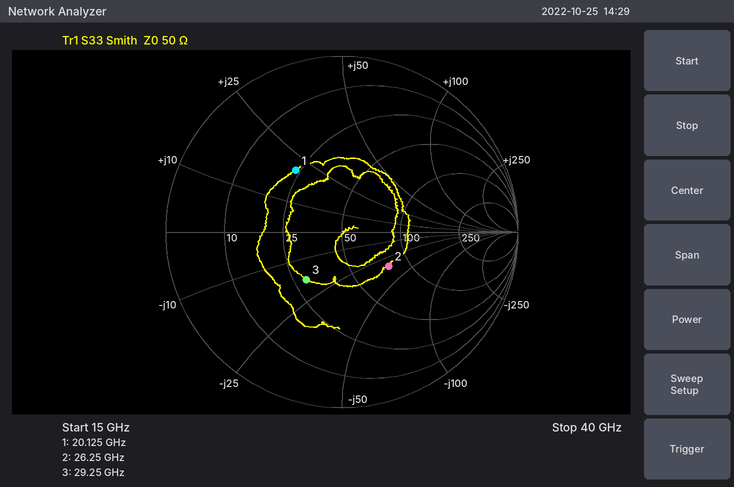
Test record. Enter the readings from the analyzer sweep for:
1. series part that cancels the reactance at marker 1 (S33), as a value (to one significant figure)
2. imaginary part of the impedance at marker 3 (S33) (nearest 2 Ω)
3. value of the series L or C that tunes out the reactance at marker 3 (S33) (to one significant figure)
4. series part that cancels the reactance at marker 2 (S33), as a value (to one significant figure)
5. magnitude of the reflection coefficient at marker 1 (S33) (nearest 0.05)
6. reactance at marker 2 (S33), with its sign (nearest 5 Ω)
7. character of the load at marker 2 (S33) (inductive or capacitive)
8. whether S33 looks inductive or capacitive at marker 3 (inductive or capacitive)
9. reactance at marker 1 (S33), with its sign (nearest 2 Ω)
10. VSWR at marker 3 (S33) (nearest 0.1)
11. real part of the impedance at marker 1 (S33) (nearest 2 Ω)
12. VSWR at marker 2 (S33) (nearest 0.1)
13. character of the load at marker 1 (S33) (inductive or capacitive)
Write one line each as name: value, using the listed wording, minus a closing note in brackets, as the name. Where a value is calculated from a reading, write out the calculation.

series part that cancels the reactance at marker 1 (S33), as a value: C = 1/(2π × 20.125 GHz × 20 Ω) ≈ 395 fF, so 400 fF to one significant figure
imaginary part of the impedance at marker 3 (S33): -18 Ω
value of the series L or C that tunes out the reactance at marker 3 (S33): L = 18 Ω/(2π × 29.25 GHz) ≈ 97.9 pH, so 100 pH to one significant figure
series part that cancels the reactance at marker 2 (S33), as a value: L = 35 Ω/(2π × 26.25 GHz) ≈ 212 pH, so 200 pH to one significant figure
magnitude of the reflection coefficient at marker 1 (S33): 0.45
reactance at marker 2 (S33), with its sign: -35 Ω
character of the load at marker 2 (S33): capacitive
whether S33 looks inductive or capacitive at marker 3: capacitive
reactance at marker 1 (S33), with its sign: +20 Ω
VSWR at marker 3 (S33): 2.0
real part of the impedance at marker 1 (S33): 24 Ω
VSWR at marker 2 (S33): 2.0
character of the load at marker 1 (S33): inductive
